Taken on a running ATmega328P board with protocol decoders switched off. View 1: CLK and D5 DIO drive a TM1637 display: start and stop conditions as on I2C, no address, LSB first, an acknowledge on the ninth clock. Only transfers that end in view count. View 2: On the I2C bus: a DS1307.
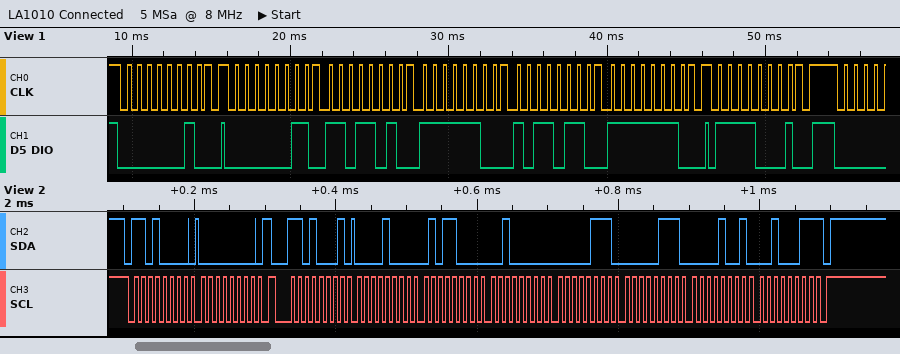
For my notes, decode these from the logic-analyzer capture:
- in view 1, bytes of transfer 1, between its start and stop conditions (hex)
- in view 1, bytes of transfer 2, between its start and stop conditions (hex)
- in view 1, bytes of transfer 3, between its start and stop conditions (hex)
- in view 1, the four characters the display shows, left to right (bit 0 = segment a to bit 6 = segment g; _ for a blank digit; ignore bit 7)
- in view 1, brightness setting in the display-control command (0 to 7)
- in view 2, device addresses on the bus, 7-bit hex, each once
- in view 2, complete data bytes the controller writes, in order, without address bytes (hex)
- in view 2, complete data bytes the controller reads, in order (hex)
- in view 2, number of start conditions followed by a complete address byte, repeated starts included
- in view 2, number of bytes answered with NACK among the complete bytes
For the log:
40
C0 5B 3F 6D 7F
8F
2058
7
0x68
00
08 58 20 07 07 09 23
2
1
